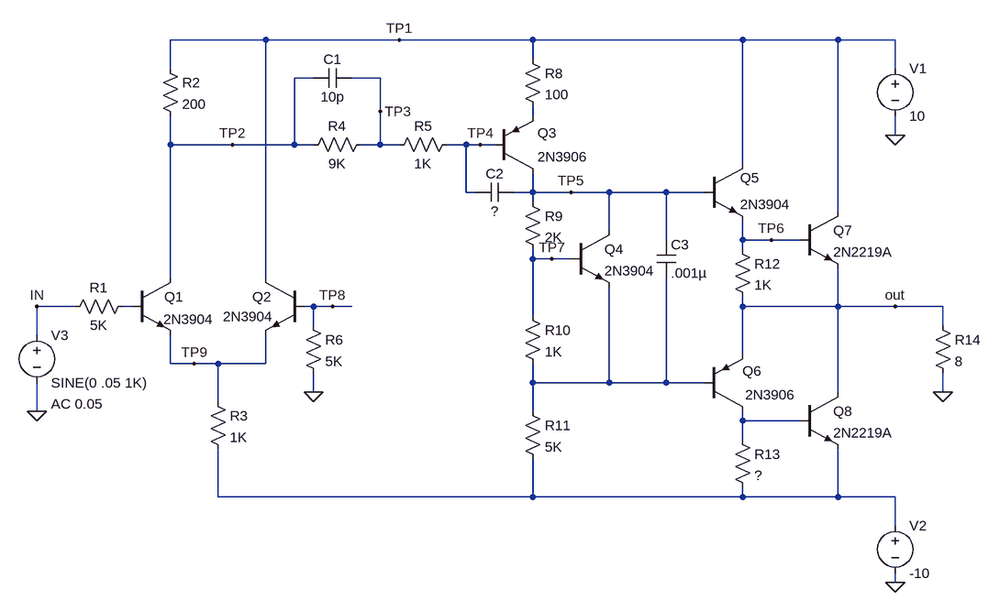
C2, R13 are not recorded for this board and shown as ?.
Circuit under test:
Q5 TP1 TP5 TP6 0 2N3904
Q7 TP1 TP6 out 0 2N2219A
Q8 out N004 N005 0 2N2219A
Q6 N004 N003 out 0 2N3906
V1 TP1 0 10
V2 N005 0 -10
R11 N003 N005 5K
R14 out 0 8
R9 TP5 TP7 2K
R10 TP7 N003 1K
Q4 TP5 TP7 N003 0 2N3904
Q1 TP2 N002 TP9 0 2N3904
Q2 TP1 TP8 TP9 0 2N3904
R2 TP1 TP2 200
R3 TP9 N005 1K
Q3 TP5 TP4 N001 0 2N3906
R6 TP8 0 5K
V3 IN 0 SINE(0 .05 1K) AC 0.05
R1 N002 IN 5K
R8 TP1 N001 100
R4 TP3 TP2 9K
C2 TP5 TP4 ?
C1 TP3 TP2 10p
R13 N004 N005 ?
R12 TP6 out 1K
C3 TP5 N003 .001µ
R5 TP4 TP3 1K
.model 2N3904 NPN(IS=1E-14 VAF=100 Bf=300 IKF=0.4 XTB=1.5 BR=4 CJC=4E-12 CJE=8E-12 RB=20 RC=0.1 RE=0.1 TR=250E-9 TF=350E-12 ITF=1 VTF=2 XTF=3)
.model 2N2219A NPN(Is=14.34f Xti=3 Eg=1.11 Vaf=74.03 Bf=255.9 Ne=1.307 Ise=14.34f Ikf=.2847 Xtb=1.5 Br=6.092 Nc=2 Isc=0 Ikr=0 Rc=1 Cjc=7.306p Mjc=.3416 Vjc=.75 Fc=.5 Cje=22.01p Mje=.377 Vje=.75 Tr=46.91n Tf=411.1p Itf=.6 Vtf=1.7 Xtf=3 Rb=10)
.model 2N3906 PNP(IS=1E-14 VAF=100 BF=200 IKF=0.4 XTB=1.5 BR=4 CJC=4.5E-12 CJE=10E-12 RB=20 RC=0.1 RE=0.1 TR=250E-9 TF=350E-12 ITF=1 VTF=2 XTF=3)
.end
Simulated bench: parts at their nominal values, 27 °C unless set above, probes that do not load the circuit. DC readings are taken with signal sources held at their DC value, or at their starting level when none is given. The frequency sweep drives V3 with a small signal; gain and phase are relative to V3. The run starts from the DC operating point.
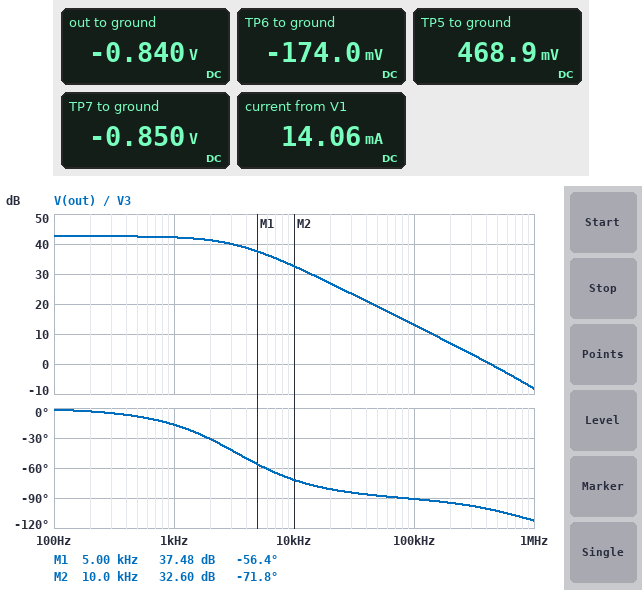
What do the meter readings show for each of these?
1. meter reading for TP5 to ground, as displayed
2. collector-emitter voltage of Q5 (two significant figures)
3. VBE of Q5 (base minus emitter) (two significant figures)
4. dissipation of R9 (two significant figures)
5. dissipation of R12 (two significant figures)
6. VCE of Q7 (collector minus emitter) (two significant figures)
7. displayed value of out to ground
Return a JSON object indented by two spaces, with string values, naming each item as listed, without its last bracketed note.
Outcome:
{
  "meter reading for TP5 to ground, as displayed": "468.9 mV",
  "collector-emitter voltage of Q5": "10 V",
  "VBE of Q5 (base minus emitter)": "640 mV",
  "dissipation of R9": "870 µW",
  "dissipation of R12": "440 µW",
  "VCE of Q7 (collector minus emitter)": "11 V",
  "displayed value of out to ground": "-0.840 V"
}
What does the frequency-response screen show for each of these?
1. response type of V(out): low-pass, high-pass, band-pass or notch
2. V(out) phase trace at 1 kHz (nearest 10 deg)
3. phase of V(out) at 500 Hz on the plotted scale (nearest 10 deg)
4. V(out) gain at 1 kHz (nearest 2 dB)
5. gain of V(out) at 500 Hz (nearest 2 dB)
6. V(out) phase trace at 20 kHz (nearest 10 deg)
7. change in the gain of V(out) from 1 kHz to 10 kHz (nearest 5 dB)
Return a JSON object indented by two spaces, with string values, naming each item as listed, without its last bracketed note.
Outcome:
{
  "response type of V(out): low-pass, high-pass, band-pass or notch": "low-pass",
  "V(out) phase trace at 1 kHz": "-20 deg",
  "phase of V(out) at 500 Hz on the plotted scale": "-10 deg",
  "V(out) gain at 1 kHz": "42 dB",
  "gain of V(out) at 500 Hz": "42 dB",
  "V(out) phase trace at 20 kHz": "-80 deg",
  "change in the gain of V(out) from 1 kHz to 10 kHz": "-10 dB"
}
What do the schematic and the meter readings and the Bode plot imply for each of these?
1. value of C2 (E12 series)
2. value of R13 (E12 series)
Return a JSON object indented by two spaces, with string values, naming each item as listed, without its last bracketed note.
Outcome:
{
  "value of C2": "150 pF",
  "value of R13": "820 Ω"
}
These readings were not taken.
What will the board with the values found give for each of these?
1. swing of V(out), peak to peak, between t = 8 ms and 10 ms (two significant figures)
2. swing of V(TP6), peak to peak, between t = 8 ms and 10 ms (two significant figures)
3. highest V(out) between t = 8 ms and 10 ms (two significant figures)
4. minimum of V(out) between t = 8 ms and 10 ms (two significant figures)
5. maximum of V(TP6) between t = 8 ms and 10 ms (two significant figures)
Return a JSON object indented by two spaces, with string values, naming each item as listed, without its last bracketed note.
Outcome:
{
  "swing of V(out), peak to peak, between t = 8 ms and 10 ms": "12 V",
  "swing of V(TP6), peak to peak, between t = 8 ms and 10 ms": "13 V",
  "highest V(out) between t = 8 ms and 10 ms": "5.4 V",
  "minimum of V(out) between t = 8 ms and 10 ms": "-6.7 V",
  "maximum of V(TP6) between t = 8 ms and 10 ms": "6.3 V"
}
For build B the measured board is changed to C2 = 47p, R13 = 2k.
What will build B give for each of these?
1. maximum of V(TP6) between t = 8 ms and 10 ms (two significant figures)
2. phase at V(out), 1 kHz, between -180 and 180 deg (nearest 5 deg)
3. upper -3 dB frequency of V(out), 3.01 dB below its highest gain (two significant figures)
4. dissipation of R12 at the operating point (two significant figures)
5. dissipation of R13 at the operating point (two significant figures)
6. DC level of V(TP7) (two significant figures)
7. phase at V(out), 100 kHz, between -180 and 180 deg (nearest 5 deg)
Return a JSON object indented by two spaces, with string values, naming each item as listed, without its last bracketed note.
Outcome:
{
  "maximum of V(TP6) between t = 8 ms and 10 ms": "6.6 V",
  "phase at V(out), 1 kHz, between -180 and 180 deg": "-5 deg",
  "upper -3 dB frequency of V(out), 3.01 dB below its highest gain": "10 kHz",
  "dissipation of R12 at the operating point": "460 µW",
  "dissipation of R13 at the operating point": "300 µW",
  "DC level of V(TP7)": "-860 mV",
  "phase at V(out), 100 kHz, between -180 and 180 deg": "-85 deg"
}
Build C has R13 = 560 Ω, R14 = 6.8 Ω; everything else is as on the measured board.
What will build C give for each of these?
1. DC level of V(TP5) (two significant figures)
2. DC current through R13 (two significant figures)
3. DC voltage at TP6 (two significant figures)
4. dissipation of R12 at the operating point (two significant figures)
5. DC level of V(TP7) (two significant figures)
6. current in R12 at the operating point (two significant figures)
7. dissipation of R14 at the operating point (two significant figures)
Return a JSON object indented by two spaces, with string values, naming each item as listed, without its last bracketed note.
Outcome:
{
  "DC level of V(TP5)": "480 mV",
  "DC current through R13": "1.4 mA",
  "DC voltage at TP6": "-160 mV",
  "dissipation of R12 at the operating point": "430 µW",
  "DC level of V(TP7)": "-840 mV",
  "current in R12 at the operating point": "660 µA",
  "dissipation of R14 at the operating point": "99 mW"
}
